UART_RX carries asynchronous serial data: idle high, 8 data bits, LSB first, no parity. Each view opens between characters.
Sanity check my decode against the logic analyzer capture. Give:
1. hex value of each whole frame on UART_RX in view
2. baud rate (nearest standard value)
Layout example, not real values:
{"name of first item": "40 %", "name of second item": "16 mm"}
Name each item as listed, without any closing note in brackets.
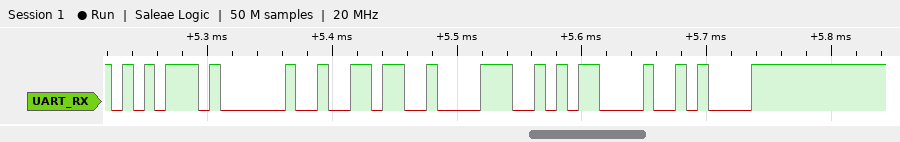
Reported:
{"hex value of each whole frame on UART_RX in view": "75, 20, 36, 38, 0D, 0A", "baud rate": "115200 baud"}
